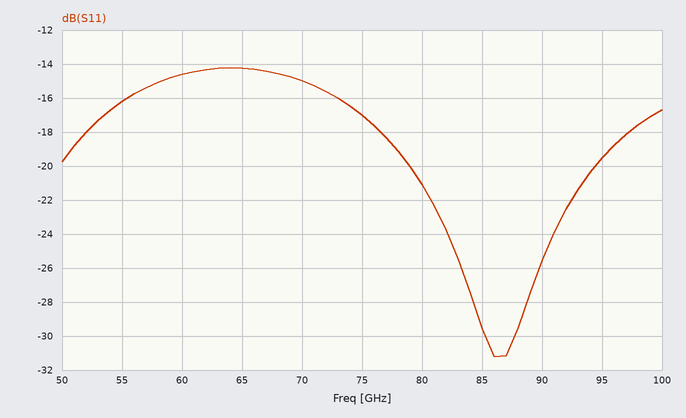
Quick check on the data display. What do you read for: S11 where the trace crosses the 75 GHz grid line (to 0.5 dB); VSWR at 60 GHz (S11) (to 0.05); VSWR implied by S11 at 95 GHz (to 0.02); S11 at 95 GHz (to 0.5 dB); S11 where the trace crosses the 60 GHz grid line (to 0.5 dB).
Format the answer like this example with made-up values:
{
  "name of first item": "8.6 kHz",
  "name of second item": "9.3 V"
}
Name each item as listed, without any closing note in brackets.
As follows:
{
  "S11 where the trace crosses the 75 GHz grid line": "-17.0 dB",
  "VSWR at 60 GHz (S11)": "1.45",
  "VSWR implied by S11 at 95 GHz": "1.24",
  "S11 at 95 GHz": "-19.5 dB",
  "S11 where the trace crosses the 60 GHz grid line": "-14.5 dB"
}
